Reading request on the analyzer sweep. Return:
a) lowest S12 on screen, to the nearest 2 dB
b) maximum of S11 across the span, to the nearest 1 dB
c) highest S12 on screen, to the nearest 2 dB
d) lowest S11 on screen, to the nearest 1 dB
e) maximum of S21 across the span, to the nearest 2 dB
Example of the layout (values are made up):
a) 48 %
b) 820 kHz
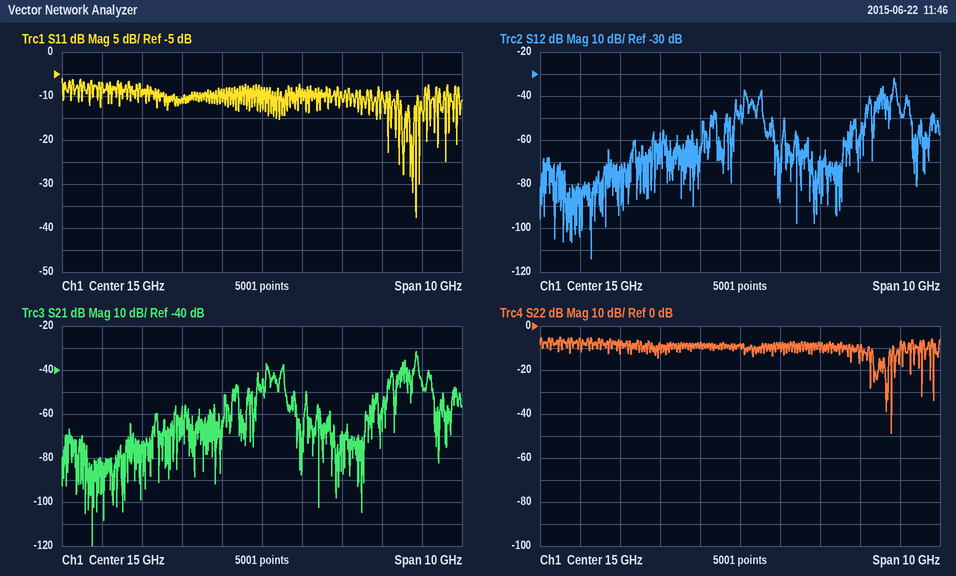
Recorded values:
a) -114 dB
b) -6 dB
c) -32 dB
d) -38 dB
e) -32 dB
